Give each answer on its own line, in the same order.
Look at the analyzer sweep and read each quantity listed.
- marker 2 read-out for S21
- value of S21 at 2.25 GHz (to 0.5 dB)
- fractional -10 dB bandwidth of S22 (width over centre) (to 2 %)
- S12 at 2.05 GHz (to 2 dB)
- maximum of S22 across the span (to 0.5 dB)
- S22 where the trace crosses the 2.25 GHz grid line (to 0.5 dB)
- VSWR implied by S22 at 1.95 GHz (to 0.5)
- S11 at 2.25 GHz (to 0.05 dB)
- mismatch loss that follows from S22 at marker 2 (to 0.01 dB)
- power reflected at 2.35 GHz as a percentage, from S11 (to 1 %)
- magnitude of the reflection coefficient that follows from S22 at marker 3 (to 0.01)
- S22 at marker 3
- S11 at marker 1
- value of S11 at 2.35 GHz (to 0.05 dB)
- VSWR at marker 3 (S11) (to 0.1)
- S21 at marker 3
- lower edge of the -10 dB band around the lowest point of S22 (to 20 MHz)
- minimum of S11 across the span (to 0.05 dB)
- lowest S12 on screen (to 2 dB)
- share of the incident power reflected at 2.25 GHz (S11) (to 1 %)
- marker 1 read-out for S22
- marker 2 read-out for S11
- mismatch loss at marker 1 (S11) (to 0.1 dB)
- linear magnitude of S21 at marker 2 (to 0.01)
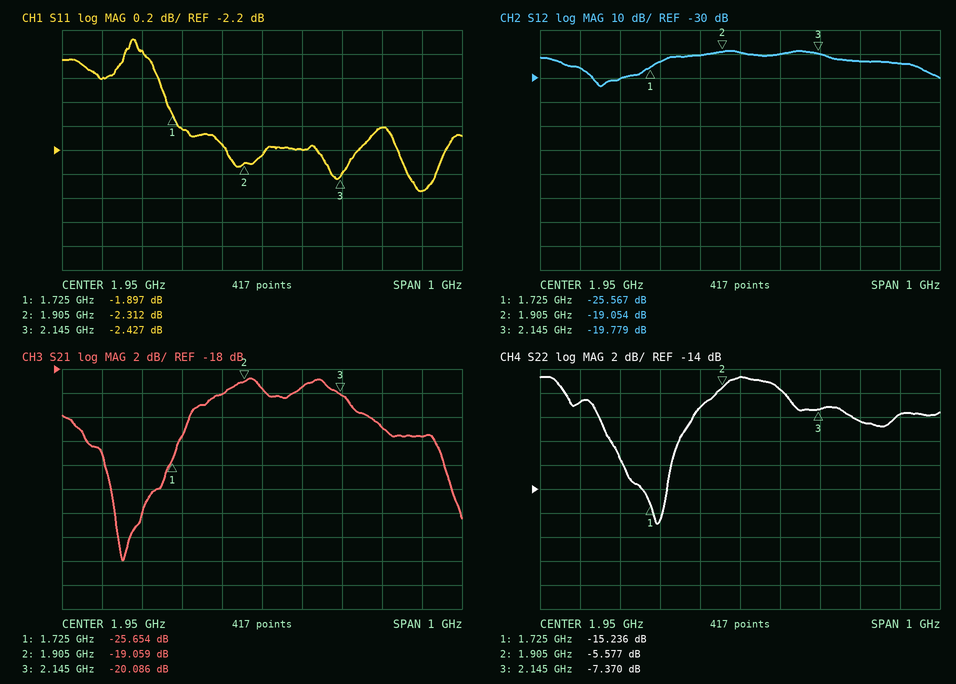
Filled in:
-19.059 dB
-23.0 dB
10 %
-20 dB
-4.5 dB
-8.5 dB
4.0
-2.00 dB
1.41 dB
56 %
0.43
-7.370 dB
-1.897 dB
-2.55 dB
7.2
-20.086 dB
1.62 GHz
-2.55 dB
-34 dB
63 %
-15.236 dB
-2.312 dB
4.5 dB
0.11
